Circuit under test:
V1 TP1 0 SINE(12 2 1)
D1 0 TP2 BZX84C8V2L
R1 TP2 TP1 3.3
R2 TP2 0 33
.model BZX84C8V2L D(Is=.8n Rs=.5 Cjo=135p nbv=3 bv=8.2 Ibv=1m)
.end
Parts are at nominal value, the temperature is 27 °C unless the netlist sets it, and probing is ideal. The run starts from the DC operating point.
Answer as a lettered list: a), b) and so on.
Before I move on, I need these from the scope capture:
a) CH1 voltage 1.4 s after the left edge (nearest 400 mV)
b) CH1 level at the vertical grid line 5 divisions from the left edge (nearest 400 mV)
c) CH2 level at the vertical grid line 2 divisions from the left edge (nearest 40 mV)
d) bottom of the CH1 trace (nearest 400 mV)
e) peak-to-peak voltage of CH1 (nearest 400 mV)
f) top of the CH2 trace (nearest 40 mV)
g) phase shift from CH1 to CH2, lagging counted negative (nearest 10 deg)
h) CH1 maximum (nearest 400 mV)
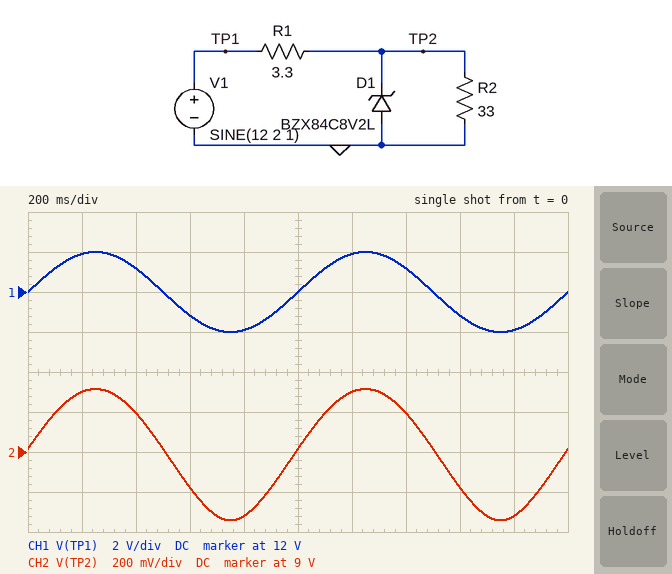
a) 13.2 V
b) 12.0 V
c) 9.20 V
d) 10.0 V
e) 4.0 V
f) 9.32 V
g) 0 deg
h) 14.0 V
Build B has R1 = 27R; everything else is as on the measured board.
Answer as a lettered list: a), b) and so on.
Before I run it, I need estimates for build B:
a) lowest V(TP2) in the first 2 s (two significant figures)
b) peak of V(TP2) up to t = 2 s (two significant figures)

a) 5.5 V
b) 7.7 V
